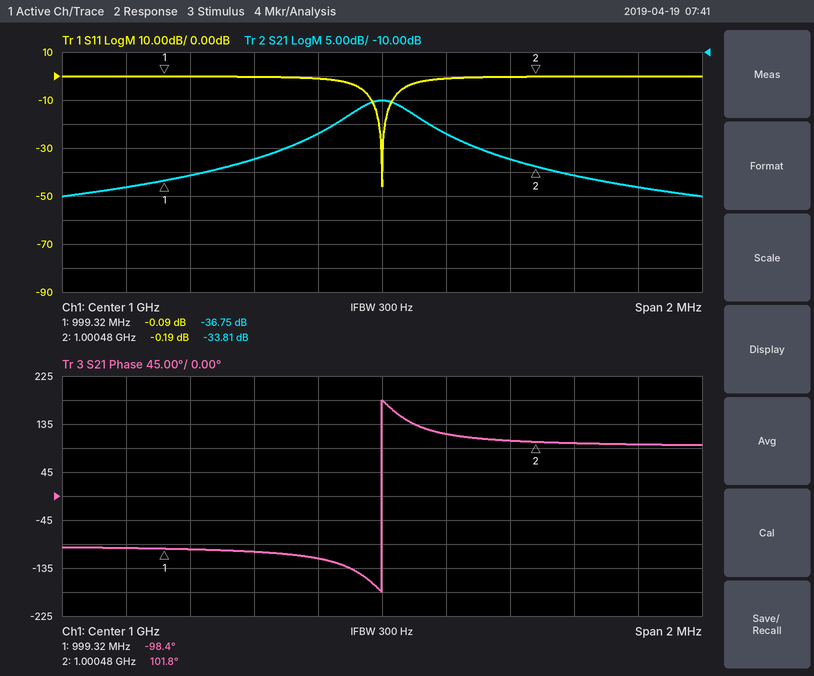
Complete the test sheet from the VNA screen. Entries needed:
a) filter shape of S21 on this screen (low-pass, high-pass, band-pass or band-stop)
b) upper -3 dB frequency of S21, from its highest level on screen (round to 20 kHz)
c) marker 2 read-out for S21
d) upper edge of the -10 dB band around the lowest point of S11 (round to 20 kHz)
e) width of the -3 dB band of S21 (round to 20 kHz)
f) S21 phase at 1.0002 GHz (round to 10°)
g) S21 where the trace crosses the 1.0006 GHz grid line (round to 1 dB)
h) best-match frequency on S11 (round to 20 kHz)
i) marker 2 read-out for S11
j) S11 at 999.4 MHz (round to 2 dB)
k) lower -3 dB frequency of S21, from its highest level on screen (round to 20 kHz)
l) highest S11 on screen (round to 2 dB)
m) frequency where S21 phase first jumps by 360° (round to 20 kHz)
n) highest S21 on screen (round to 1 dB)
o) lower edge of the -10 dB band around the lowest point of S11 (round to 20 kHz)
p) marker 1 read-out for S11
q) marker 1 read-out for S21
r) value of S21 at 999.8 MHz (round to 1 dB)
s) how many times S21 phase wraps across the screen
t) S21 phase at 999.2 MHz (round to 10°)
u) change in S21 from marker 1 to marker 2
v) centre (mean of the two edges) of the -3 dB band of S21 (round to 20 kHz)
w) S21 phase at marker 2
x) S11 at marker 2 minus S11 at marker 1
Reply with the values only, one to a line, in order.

band-pass
1.00010 GHz
-33.81 dB
1.00004 GHz
200 kHz
120°
-36 dB
1.00000 GHz
-0.19 dB
0 dB
999.90 MHz
0 dB
1.00000 GHz
-20 dB
999.96 MHz
-0.09 dB
-36.75 dB
-27 dB
1
-100°
2.94 dB
1.00000 GHz
101.8°
-0.10 dB
